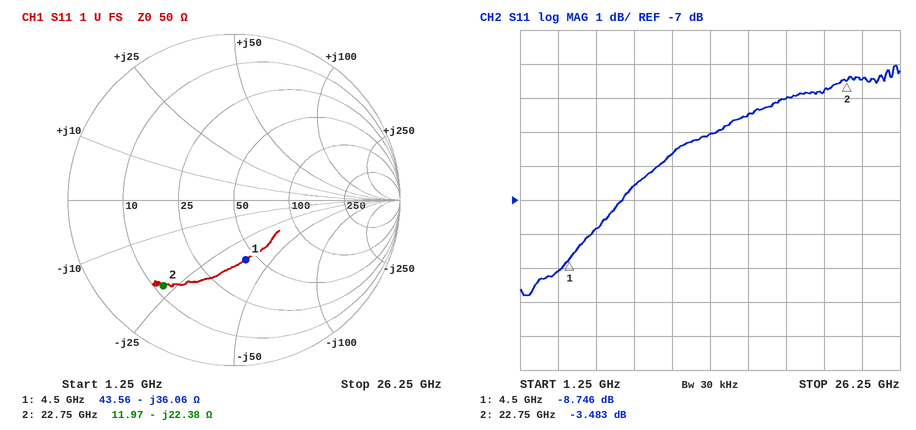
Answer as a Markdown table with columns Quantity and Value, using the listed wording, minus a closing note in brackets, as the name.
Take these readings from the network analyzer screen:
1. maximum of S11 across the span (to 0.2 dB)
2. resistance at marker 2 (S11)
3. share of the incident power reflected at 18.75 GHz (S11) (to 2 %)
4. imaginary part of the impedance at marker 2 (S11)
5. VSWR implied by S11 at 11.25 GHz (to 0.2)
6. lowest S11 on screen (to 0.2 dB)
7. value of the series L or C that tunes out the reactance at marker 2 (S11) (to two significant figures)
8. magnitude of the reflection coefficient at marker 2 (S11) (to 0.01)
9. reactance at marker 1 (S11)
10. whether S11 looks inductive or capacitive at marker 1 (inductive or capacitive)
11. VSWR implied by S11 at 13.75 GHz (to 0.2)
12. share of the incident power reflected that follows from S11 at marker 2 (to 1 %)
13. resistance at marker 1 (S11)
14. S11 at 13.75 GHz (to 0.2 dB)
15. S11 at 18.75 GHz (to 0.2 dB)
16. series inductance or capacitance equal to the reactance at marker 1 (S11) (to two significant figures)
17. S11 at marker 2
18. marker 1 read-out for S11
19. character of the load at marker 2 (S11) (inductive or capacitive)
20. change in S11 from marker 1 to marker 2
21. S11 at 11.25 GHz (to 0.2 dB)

| Quantity | Value |
|---|---|
| maximum of S11 across the span | -3.0 dB |
| resistance at marker 2 | 11.97 Ω |
| share of the incident power reflected at 18.75 GHz (S11) | 40 % |
| imaginary part of the impedance at marker 2 | -22.38 Ω |
| VSWR implied by S11 at 11.25 GHz | 3.2 |
| lowest S11 on screen | -9.8 dB |
| value of the series L or C that tunes out the reactance at marker 2 (S11) | 160 pH |
| magnitude of the reflection coefficient at marker 2 (S11) | 0.67 |
| reactance at marker 1 | -36.06 Ω |
| whether S11 looks inductive or capacitive at marker 1 | capacitive |
| VSWR implied by S11 at 13.75 GHz | 3.6 |
| share of the incident power reflected that follows from S11 at marker 2 | 45 % |
| resistance at marker 1 | 43.56 Ω |
| S11 at 13.75 GHz | -5.0 dB |
| S11 at 18.75 GHz | -4.0 dB |
| series inductance or capacitance equal to the reactance at marker 1 (S11) | 980 fF |
| S11 at marker 2 | -3.483 dB |
| marker 1 read-out for S11 | -8.746 dB |
| character of the load at marker 2 (S11) | capacitive |
| change in S11 from marker 1 to marker 2 | 5.263 dB |
| S11 at 11.25 GHz | -5.6 dB |
